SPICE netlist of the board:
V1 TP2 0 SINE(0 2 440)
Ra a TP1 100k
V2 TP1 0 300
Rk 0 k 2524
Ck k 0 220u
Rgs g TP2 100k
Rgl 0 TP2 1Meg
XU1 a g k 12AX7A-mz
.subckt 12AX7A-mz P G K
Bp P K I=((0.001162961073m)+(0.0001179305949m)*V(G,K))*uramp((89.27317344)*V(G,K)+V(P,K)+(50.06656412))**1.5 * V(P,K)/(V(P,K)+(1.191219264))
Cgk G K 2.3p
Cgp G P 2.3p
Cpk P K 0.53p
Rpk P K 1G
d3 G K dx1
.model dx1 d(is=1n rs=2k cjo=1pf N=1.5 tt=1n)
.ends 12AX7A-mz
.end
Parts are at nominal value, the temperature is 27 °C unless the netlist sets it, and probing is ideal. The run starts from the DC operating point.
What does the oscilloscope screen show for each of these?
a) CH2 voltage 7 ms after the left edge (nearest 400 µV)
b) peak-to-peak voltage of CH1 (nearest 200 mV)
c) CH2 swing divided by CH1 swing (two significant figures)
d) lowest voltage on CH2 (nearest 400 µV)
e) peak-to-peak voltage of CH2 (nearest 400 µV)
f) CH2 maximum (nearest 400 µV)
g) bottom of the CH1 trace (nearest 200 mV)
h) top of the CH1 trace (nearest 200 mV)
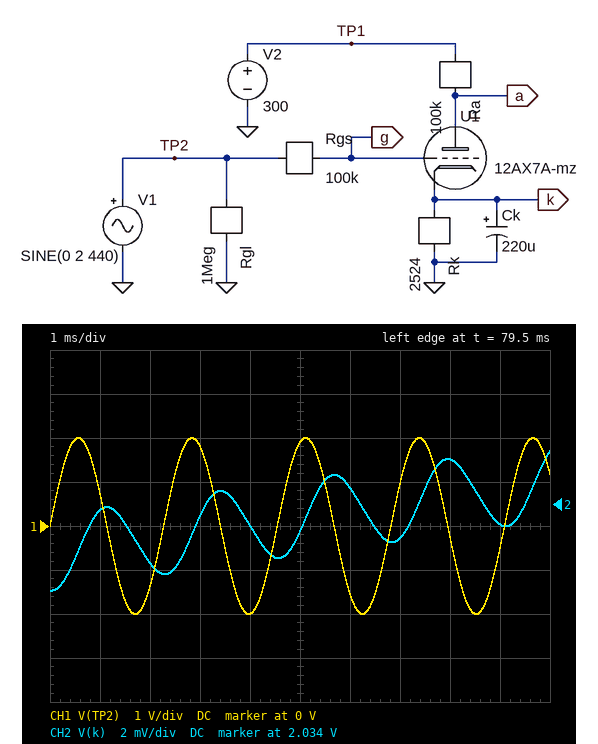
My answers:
2.0324 V
4.0 V
0.0016
2.0300 V
6.4 mV
2.0364 V
-2.0 V
2.0 V
